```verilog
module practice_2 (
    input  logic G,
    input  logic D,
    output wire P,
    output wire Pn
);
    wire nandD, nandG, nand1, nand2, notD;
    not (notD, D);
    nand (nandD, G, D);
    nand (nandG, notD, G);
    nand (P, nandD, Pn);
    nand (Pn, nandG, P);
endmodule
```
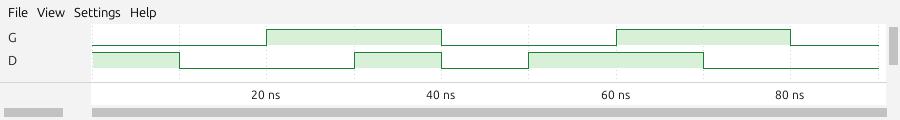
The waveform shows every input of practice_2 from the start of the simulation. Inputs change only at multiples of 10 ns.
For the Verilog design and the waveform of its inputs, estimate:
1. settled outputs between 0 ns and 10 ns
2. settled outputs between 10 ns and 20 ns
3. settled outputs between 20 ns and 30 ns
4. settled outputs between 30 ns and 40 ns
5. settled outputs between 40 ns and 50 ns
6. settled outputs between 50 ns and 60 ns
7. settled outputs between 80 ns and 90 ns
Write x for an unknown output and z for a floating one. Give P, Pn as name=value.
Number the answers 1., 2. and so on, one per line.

1. P=x, Pn=x
2. P=x, Pn=x
3. P=0, Pn=1
4. P=1, Pn=0
5. P=1, Pn=0
6. P=1, Pn=0
7. P=0, Pn=1
